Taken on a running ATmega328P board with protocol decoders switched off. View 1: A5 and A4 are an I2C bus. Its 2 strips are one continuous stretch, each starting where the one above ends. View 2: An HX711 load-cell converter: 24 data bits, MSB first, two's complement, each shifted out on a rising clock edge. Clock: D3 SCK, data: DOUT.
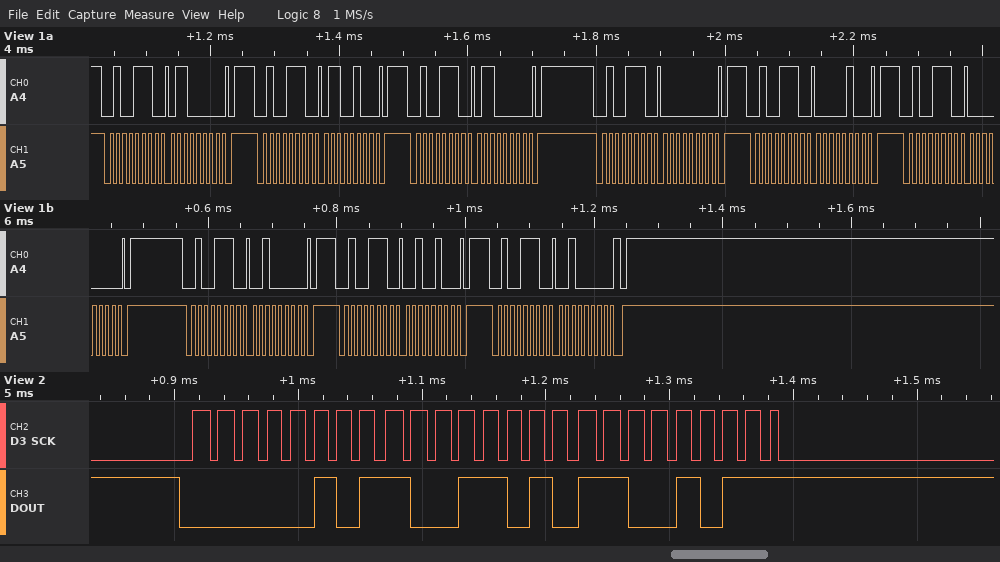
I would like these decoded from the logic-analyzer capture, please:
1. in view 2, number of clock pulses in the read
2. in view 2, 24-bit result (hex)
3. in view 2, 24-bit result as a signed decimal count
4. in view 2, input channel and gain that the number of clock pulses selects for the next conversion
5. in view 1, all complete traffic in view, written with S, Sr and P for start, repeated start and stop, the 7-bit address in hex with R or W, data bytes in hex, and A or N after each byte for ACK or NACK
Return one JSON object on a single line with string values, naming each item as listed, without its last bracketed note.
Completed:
{"in view 2, number of clock pulses in the read": "25", "in view 2, 24-bit result": "0x059ACB", "in view 2, 24-bit result as a signed decimal count": "367307", "in view 2, input channel and gain that the number of clock pulses selects for the next conversion": "channel A, gain 128", "in view 1, all complete traffic in view, written with S, Sr and P for start, repeated start and stop, the 7-bit address in hex with R or W, data bytes in hex, and A or N after each byte for ACK or NACK": "S 27W A 60 A P S 27W A 64 A P S 27W A 60 A P S 27W A 00 A P S 27W A 04 A P S 27W A 00 A P S 27W A 20 A P S 27W A 24 A P S 27W A 20 A P"}
